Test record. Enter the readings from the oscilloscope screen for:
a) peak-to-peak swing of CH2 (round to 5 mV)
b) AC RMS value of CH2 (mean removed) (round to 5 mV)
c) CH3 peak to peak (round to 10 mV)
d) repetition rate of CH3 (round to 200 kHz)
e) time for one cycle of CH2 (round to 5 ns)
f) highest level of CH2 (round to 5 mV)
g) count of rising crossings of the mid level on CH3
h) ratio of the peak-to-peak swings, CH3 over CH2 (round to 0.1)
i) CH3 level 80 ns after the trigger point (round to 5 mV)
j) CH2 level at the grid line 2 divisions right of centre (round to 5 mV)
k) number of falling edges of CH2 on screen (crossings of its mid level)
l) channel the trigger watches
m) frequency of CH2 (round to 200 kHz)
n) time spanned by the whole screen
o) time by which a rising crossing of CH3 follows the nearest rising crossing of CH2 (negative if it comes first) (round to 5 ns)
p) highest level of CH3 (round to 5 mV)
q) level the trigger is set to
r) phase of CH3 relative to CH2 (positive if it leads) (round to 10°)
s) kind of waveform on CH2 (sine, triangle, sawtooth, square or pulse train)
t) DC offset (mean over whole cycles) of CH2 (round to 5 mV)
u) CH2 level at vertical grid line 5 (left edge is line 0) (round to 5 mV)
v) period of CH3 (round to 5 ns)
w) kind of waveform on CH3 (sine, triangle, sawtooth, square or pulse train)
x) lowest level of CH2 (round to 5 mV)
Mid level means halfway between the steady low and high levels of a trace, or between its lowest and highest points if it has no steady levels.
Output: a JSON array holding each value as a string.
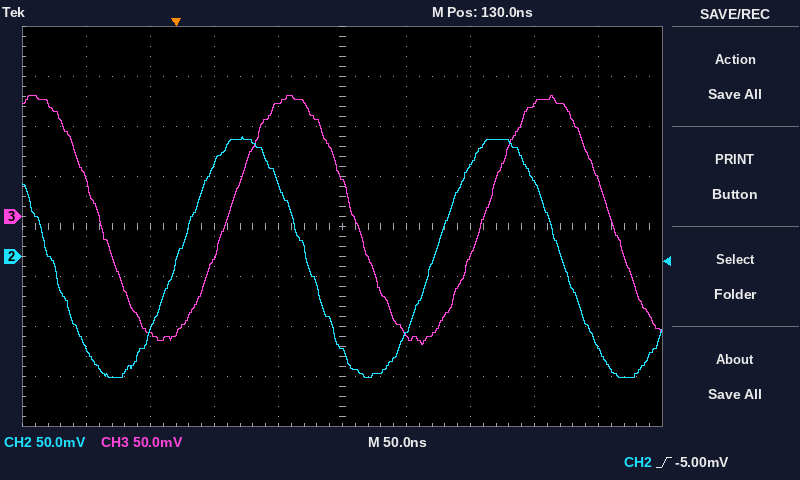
["240 mV", "85 mV", "250 mV", "5.0 MHz", "200 ns", "120 mV", "2", "1.0", "115 mV", "90 mV", "3", "CH2", "5.0 MHz", "500 ns", "+40 ns", "120 mV", "-5.00 mV", "-70°", "sine", "0 mV", "-95 mV", "200 ns", "sine", "-120 mV"]
